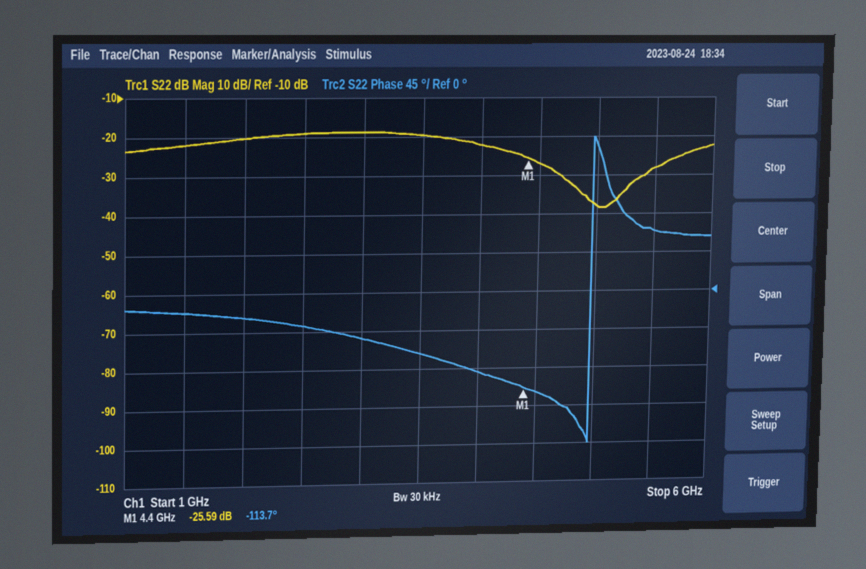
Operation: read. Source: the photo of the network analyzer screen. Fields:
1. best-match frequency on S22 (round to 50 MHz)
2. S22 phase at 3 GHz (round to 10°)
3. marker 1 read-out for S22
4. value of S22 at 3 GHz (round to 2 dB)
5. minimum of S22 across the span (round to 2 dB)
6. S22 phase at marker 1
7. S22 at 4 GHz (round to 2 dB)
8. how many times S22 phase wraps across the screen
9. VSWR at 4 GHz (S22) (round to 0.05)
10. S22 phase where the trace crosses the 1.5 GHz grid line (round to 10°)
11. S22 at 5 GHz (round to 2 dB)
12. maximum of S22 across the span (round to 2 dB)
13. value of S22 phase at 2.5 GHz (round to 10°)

5.00 GHz
-50°
-25.59 dB
-18 dB
-38 dB
-113.7°
-22 dB
1
1.15
-20°
-38 dB
-18 dB
-40°
